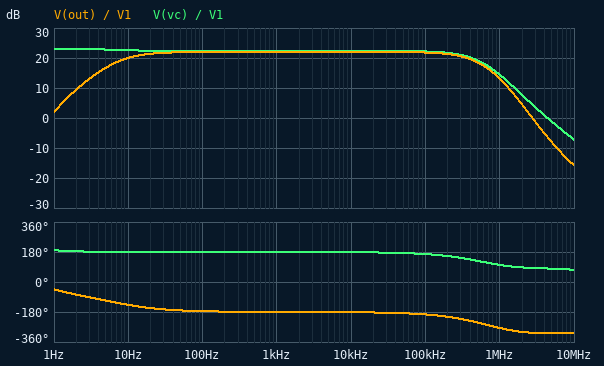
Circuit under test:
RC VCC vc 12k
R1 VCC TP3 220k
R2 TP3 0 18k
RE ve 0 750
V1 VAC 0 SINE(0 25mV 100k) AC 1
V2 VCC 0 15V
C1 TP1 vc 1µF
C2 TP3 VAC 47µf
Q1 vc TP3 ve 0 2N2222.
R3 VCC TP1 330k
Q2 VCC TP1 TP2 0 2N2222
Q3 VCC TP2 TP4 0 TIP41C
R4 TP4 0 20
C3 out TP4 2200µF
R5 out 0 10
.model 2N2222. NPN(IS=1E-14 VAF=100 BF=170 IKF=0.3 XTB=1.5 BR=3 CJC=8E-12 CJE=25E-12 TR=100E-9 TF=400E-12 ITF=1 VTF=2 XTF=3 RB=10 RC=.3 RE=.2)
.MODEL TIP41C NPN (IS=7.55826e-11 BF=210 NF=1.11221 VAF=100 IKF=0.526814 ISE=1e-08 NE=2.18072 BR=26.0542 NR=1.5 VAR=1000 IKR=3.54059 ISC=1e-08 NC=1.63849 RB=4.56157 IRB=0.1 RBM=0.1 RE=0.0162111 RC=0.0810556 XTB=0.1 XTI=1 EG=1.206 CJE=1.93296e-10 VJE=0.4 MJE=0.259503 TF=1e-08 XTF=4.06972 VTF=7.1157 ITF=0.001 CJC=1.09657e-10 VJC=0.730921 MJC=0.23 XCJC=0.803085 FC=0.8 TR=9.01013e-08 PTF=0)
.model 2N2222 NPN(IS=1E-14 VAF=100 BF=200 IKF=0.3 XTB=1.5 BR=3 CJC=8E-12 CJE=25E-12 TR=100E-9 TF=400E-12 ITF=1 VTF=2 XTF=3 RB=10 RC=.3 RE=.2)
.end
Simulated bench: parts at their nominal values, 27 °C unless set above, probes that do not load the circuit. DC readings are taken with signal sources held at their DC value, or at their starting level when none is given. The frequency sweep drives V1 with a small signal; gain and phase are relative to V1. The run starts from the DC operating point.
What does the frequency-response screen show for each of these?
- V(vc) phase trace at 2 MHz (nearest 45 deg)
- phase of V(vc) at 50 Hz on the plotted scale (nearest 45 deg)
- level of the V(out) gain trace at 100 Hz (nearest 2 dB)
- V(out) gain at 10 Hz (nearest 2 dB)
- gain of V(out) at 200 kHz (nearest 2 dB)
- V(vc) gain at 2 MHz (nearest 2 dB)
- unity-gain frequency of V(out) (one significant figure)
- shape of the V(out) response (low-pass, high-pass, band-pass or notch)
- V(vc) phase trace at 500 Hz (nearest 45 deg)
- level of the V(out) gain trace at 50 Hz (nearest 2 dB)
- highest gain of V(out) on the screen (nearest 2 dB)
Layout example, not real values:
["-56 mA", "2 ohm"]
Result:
["90 deg", "180 deg", "22 dB", "20 dB", "22 dB", "8 dB", "3 MHz", "band-pass", "180 deg", "22 dB", "22 dB"]
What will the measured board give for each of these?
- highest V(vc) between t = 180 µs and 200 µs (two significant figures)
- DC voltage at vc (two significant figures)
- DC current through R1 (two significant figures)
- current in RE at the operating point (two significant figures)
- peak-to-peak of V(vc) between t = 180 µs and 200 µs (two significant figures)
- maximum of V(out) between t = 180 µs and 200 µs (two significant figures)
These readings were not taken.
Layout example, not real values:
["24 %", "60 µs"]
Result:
["8.3 V", "8.0 V", "63 µA", "590 µA", "640 mV", "310 mV"]
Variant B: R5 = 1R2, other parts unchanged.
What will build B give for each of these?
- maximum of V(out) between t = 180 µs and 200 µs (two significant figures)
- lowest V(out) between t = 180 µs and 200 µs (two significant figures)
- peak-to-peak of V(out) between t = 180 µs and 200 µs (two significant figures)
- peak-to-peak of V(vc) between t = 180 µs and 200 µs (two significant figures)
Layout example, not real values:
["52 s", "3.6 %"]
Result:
["160 mV", "-160 mV", "330 mV", "410 mV"]
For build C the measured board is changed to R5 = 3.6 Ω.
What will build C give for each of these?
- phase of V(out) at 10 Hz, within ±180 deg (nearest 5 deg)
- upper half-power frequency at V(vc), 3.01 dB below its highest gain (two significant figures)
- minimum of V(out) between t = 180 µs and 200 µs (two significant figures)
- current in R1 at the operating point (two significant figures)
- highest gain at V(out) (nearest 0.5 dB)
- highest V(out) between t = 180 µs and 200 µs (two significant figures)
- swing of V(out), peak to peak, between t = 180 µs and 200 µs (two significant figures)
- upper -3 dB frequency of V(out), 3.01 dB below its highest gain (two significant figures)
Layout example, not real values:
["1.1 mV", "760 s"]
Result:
["-115 deg", "190 kHz", "-260 mV", "63 µA", "21.0 dB", "260 mV", "520 mV", "280 kHz"]
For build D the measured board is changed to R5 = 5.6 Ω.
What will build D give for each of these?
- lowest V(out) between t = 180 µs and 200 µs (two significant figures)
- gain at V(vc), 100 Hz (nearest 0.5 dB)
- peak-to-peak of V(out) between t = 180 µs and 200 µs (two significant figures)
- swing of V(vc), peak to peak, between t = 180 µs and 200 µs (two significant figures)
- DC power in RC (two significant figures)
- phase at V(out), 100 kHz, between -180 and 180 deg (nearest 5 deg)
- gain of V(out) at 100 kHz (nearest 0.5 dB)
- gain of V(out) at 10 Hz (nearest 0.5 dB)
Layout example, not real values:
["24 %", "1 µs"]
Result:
["-290 mV", "22.0 dB", "570 mV", "610 mV", "4.1 mW", "160 deg", "21.0 dB", "17.5 dB"]
